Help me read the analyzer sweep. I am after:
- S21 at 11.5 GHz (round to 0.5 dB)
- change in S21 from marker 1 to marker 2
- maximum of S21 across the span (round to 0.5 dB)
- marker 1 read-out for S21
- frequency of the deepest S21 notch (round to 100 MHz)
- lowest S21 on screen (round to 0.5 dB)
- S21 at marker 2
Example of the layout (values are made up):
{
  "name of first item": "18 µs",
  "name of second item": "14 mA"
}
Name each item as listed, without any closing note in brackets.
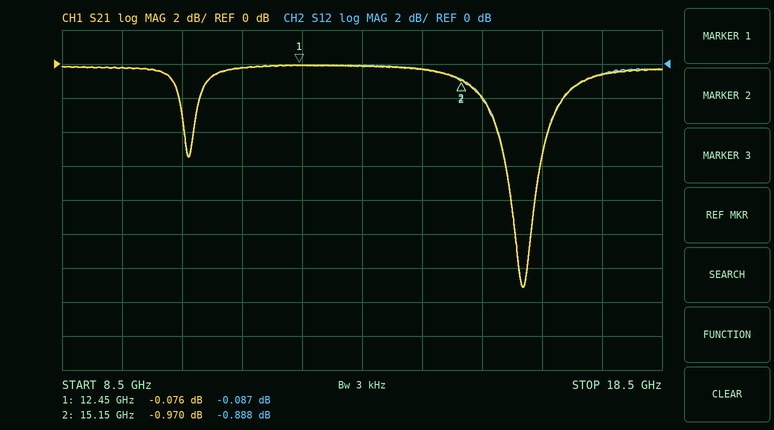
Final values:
{
  "S21 at 11.5 GHz": "0.0 dB",
  "change in S21 from marker 1 to marker 2": "-0.894 dB",
  "maximum of S21 across the span": "0.0 dB",
  "marker 1 read-out for S21": "-0.076 dB",
  "frequency of the deepest S21 notch": "16.2 GHz",
  "lowest S21 on screen": "-13.0 dB",
  "S21 at marker 2": "-0.970 dB"
}
